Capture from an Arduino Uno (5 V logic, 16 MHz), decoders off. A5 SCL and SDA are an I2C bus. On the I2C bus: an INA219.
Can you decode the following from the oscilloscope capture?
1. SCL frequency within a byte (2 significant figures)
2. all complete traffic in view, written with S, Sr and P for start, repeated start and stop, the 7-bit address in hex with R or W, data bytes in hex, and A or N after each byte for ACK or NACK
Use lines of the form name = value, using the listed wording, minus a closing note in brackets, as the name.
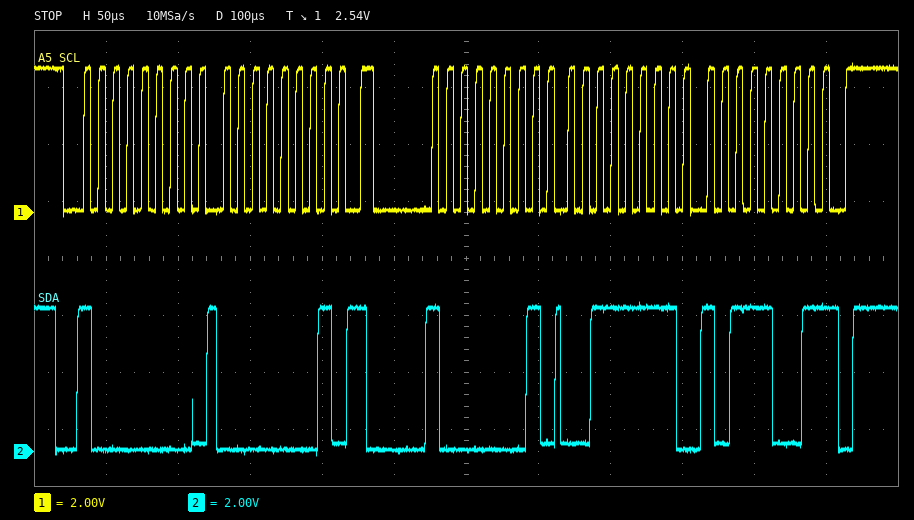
SCL frequency within a byte = 100 kHz
all complete traffic in view, written with S, Sr and P for start, repeated start and stop, the 7-bit address in hex with R or W, data bytes in hex, and A or N after each byte for ACK or NACK = S 40W A 01 A Sr 40R A 3F A B9 N P
